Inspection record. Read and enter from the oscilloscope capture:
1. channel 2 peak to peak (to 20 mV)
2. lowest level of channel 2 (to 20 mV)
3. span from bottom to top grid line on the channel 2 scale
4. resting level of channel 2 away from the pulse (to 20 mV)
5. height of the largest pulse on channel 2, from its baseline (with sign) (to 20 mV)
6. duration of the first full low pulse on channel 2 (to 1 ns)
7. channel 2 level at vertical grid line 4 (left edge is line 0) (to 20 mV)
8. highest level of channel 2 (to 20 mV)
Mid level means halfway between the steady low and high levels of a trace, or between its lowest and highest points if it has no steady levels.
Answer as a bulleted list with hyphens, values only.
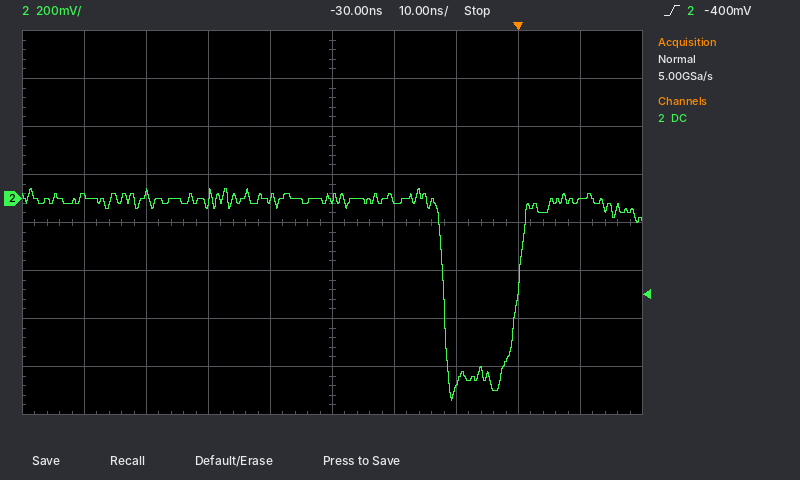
- 880 mV
- -840 mV
- 1.6 V
- 0 mV
- -840 mV
- 12 ns
- 0 mV
- 40 mV
